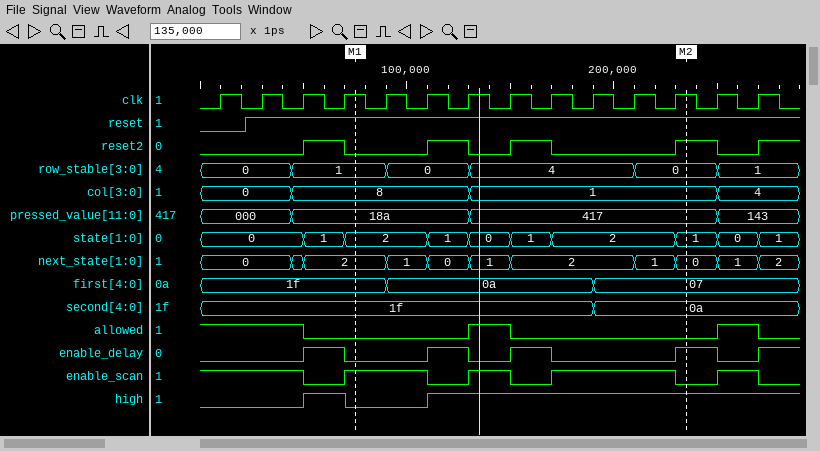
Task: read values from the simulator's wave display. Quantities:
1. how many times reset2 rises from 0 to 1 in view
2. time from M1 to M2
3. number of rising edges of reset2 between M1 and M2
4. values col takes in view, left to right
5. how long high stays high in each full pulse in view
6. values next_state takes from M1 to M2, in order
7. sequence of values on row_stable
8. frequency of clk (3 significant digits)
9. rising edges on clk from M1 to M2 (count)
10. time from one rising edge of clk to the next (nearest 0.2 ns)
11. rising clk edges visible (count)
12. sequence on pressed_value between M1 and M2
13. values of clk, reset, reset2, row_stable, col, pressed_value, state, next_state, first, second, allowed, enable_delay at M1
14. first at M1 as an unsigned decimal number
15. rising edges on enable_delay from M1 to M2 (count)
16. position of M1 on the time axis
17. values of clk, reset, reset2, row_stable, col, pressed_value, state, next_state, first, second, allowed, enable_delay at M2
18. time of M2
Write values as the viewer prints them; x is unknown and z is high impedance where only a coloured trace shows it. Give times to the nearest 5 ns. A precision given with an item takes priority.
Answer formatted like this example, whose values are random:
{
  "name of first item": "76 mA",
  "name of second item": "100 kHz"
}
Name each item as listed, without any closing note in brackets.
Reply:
{
  "how many times reset2 rises from 0 to 1 in view": "5",
  "time from M1 to M2": "160 ns",
  "number of rising edges of reset2 between M1 and M2": "3",
  "values col takes in view, left to right": "0, 8, 1, 4",
  "how long high stays high in each full pulse in view": "20 ns",
  "values next_state takes from M1 to M2, in order": "2, 1, 0, 1, 2, 1, 0",
  "sequence of values on row_stable": "0, 1, 0, 4, 0, 1",
  "frequency of clk": "50.0 MHz",
  "rising edges on clk from M1 to M2": "8",
  "time from one rising edge of clk to the next": "20 ns",
  "rising clk edges visible": "14",
  "sequence on pressed_value between M1 and M2": "18a, 417",
  "values of clk, reset, reset2, row_stable, col, pressed_value, state, next_state, first, second, allowed, enable_delay at M1": "clk=1, reset=1, reset2=0, row_stable=1, col=8, pressed_value=18a, state=2, next_state=2, first=1f, second=1f, allowed=0, enable_delay=0",
  "first at M1 as an unsigned decimal number": "31",
  "rising edges on enable_delay from M1 to M2": "3",
  "position of M1 on the time axis": "75 ns",
  "values of clk, reset, reset2, row_stable, col, pressed_value, state, next_state, first, second, allowed, enable_delay at M2": "clk=1, reset=1, reset2=1, row_stable=0, col=1, pressed_value=417, state=1, next_state=0, first=07, second=0a, allowed=0, enable_delay=1",
  "time of M2": "235 ns"
}
